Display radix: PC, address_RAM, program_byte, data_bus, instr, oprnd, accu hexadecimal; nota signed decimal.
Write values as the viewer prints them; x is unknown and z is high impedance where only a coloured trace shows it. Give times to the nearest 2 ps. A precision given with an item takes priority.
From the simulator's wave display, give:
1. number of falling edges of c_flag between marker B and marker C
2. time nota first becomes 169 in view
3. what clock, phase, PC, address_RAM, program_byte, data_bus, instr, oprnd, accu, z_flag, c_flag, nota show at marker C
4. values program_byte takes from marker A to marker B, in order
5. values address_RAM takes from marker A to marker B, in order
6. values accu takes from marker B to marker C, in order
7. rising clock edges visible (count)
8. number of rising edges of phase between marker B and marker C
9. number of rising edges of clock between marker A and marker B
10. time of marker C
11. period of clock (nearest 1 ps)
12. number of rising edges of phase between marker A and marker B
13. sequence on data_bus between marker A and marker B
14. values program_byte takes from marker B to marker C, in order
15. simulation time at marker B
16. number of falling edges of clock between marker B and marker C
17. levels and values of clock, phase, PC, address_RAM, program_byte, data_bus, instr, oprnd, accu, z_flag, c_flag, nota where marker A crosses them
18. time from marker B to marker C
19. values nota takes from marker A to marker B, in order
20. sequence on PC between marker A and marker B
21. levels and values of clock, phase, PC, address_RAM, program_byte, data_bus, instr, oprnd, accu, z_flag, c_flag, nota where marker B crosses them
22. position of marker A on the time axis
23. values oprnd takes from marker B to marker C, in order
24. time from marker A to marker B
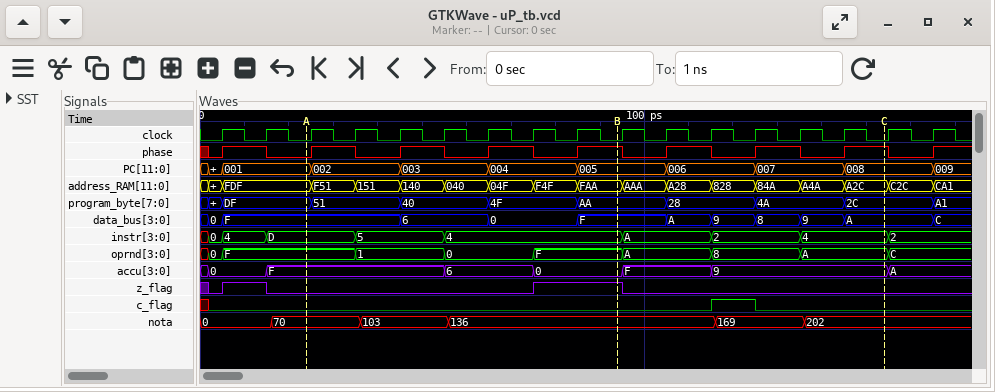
1
116 ps
clock=0, phase=1, PC=008, address_RAM=A2C, program_byte=2C, data_bus=A, instr=4, oprnd=A, accu=9, z_flag=0, c_flag=0, nota=202
DF, 51, 40, 4F, AA
FDF, F51, 151, 140, 040, 04F, F4F, FAA
0, F, 9
17
3
7
154 ps
10 ps
4
F, 6, 0, F
AA, 28, 4A, 2C
94 ps
6
clock=0, phase=0, PC=001, address_RAM=FDF, program_byte=DF, data_bus=F, instr=D, oprnd=F, accu=F, z_flag=0, c_flag=0, nota=70
60 ps
70, 103, 136
001, 002, 003, 004, 005
clock=0, phase=1, PC=005, address_RAM=FAA, program_byte=AA, data_bus=F, instr=4, oprnd=F, accu=0, z_flag=1, c_flag=0, nota=136
24 ps
F, A, 8, A
70 ps
